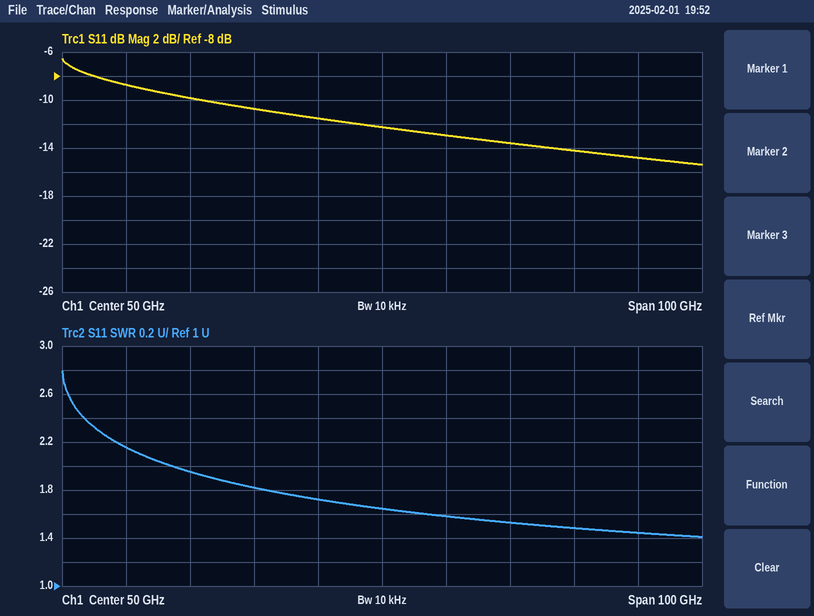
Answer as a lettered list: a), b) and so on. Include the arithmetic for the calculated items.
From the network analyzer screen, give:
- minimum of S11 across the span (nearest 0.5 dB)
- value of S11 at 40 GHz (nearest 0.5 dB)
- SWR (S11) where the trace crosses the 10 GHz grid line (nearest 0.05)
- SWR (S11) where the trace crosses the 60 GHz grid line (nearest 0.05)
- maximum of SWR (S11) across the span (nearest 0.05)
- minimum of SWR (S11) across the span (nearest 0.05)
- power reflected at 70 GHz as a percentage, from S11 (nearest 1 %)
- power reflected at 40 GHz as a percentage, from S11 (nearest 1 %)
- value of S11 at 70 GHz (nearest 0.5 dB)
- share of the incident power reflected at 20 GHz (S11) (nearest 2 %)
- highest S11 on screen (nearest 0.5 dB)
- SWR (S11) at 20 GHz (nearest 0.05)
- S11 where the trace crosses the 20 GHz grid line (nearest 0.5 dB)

a) -15.5 dB
b) -11.5 dB
c) 2.15
d) 1.60
e) 2.80
f) 1.40
g) 10^(-13.5/10) ≈ 4 %
h) 10^(-11.5/10) ≈ 7 %
i) -13.5 dB
j) 10^(-10/10) ≈ 10 %
k) -6.5 dB
l) 1.95
m) -10.0 dB
